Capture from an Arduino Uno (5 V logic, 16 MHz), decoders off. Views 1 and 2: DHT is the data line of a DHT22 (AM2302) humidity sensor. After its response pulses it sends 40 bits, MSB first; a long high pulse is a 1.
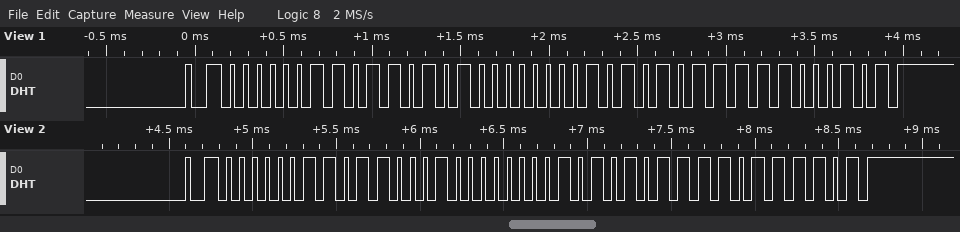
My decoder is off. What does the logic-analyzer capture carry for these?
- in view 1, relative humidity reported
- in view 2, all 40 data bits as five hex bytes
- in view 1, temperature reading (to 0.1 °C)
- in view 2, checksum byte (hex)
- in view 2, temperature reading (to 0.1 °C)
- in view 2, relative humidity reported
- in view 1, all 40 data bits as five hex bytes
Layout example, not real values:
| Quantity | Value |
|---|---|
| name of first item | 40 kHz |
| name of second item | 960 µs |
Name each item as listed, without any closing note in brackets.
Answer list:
| Quantity | Value |
|---|---|
| in view 1, relative humidity reported | 87.4 % |
| in view 2, all 40 data bits as five hex bytes | 03 62 01 57 BD |
| in view 1, temperature reading | 34.3 °C |
| in view 2, checksum byte | 0xBD |
| in view 2, temperature reading | 34.3 °C |
| in view 2, relative humidity reported | 86.6 % |
| in view 1, all 40 data bits as five hex bytes | 03 6A 01 57 C5 |
